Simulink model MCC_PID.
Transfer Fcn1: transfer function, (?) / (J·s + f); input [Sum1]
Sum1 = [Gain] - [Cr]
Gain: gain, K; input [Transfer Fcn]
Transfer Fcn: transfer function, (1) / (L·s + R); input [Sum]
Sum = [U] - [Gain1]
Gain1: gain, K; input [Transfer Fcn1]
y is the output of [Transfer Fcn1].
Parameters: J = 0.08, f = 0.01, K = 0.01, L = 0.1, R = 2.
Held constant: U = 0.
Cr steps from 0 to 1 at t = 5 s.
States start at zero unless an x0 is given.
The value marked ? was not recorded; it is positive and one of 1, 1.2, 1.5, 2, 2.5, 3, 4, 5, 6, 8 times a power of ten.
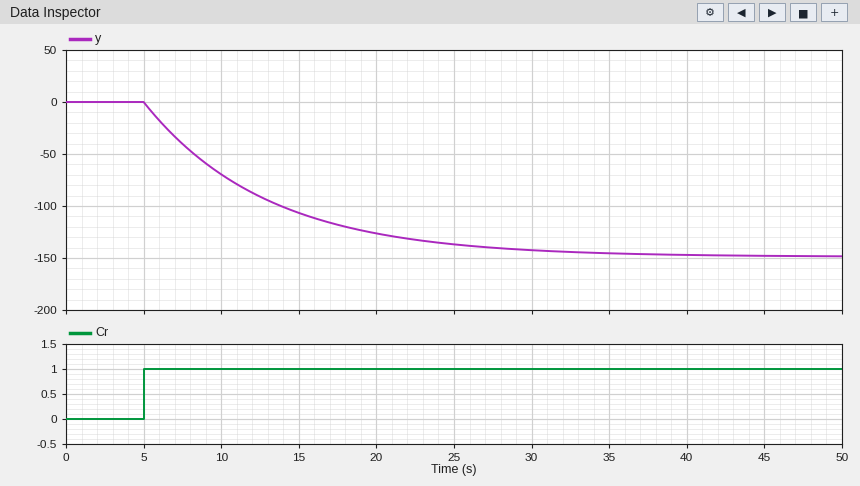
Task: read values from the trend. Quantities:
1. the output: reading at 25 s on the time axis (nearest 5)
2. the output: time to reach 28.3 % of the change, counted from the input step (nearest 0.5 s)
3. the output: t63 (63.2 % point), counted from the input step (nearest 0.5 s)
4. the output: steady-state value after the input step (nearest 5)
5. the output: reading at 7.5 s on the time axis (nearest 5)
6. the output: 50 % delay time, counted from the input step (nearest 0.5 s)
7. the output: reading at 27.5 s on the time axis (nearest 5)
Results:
-135
2.5 s
8.0 s
-150
-40
5.5 s
-140
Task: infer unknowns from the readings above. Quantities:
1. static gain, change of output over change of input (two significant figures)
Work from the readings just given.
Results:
-150
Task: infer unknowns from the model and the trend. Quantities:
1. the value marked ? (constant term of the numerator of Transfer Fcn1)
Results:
1.5
